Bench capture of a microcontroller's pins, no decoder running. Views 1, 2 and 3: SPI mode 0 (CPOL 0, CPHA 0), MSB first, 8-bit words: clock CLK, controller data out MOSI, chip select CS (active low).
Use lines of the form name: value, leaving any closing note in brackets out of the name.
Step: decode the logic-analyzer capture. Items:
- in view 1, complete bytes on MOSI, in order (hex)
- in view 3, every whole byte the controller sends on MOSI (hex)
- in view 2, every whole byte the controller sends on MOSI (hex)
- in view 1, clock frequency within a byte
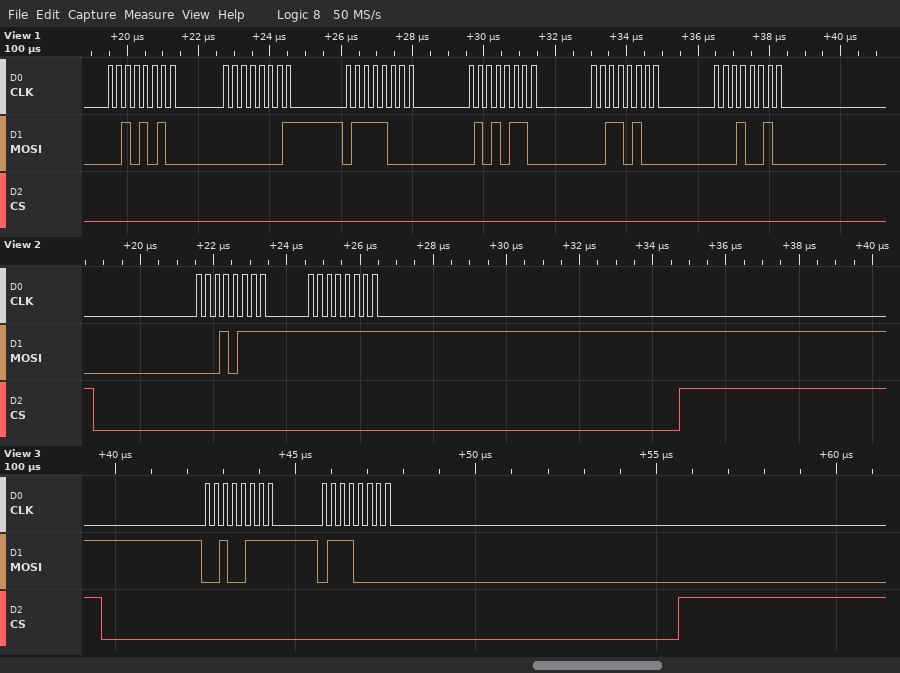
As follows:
in view 1, complete bytes on MOSI, in order: 2A 01 78 56 34 12
in view 3, every whole byte the controller sends on MOSI: 0x27 0x70
in view 2, every whole byte the controller sends on MOSI: 17 FF
in view 1, clock frequency within a byte: 4 MHz
